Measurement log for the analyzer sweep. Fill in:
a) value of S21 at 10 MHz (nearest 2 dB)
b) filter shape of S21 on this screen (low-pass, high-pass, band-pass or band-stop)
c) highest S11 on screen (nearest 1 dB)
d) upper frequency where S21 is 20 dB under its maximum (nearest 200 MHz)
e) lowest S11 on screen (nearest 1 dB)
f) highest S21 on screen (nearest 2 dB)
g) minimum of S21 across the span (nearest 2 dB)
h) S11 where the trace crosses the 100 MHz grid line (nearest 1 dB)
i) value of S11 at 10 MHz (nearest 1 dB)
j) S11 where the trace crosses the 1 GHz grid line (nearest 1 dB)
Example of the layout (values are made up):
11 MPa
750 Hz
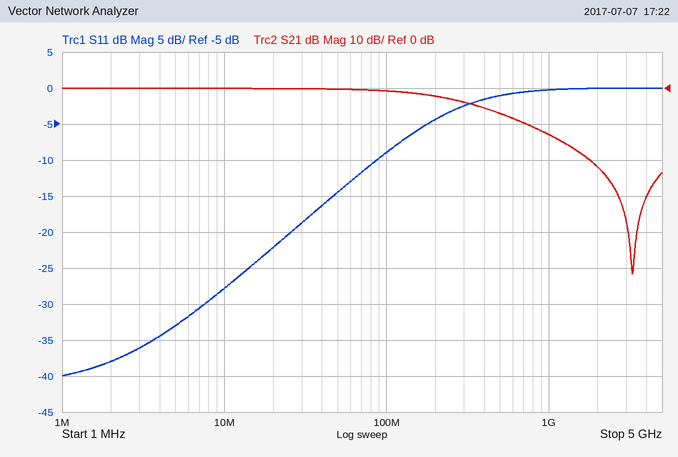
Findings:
0 dB
low-pass
0 dB
1.8 GHz
-40 dB
0 dB
-52 dB
-9 dB
-28 dB
0 dB
